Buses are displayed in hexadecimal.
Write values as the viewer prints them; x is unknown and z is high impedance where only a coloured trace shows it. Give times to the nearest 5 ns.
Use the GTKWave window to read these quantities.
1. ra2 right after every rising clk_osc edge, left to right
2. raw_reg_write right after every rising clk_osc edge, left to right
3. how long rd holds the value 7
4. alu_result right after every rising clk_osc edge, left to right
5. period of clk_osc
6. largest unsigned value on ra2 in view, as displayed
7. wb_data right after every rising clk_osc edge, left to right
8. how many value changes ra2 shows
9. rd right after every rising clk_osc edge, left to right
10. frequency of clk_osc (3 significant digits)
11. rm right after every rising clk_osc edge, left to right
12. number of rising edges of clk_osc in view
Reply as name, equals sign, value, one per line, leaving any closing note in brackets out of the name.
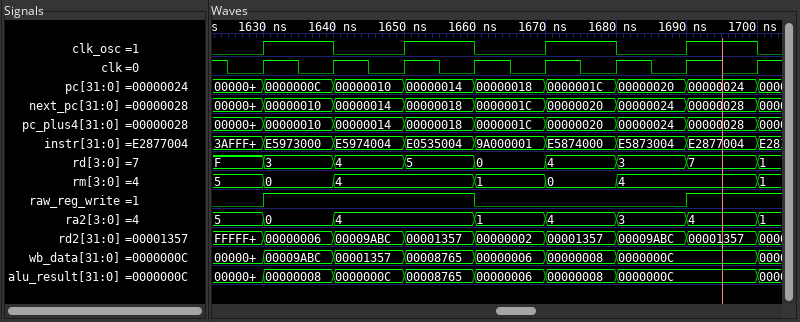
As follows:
ra2 right after every rising clk_osc edge, left to right = 0, 4, 4, 4
raw_reg_write right after every rising clk_osc edge, left to right = 1 1 0 1
how long rd holds the value 7 = 10 ns
alu_result right after every rising clk_osc edge, left to right = 00000008, 00008765, 00000008, 0000000C
period of clk_osc = 20 ns
largest unsigned value on ra2 in view, as displayed = 5
wb_data right after every rising clk_osc edge, left to right = 00009ABC, 00008765, 00000008, 0000000C
how many value changes ra2 shows = 7
rd right after every rising clk_osc edge, left to right = 3, 5, 4, 7
frequency of clk_osc = 50.0 MHz
rm right after every rising clk_osc edge, left to right = 0, 4, 0, 4
number of rising edges of clk_osc in view = 4
